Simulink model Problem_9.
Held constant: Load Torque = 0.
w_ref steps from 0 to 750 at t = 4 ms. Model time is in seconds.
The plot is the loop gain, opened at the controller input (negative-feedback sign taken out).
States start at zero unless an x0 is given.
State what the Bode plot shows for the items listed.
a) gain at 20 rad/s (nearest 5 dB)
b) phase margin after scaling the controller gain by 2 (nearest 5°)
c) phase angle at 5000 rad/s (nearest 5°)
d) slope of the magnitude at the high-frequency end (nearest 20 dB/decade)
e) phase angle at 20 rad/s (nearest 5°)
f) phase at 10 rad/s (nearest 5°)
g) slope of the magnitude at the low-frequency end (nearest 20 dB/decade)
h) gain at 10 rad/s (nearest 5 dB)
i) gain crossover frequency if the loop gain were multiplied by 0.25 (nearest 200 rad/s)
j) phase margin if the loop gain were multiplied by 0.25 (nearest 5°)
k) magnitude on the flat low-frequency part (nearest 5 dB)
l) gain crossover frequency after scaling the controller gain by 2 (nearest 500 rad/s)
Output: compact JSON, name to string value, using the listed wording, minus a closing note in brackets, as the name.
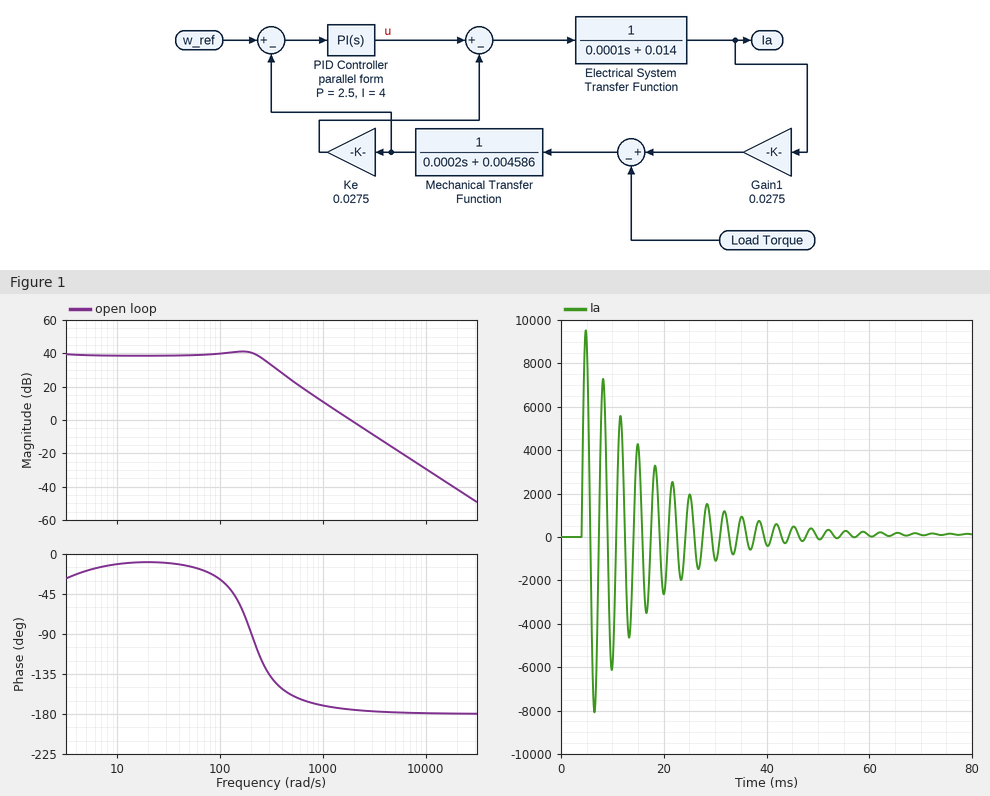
{"gain at 20 rad/s": "40 dB", "phase margin after scaling the controller gain by 2": "5°", "phase angle at 5000 rad/s": "-180°", "slope of the magnitude at the high-frequency end": "-40 dB/decade", "phase angle at 20 rad/s": "-10°", "phase at 10 rad/s": "-10°", "slope of the magnitude at the low-frequency end": "0 dB/decade", "gain at 10 rad/s": "40 dB", "gain crossover frequency if the loop gain were multiplied by 0.25": "1000 rad/s", "phase margin if the loop gain were multiplied by 0.25": "10°", "magnitude on the flat low-frequency part": "40 dB", "gain crossover frequency after scaling the controller gain by 2": "2500 rad/s"}
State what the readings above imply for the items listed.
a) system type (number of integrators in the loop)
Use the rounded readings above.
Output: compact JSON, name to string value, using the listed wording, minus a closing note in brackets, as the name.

{"system type": "0"}
